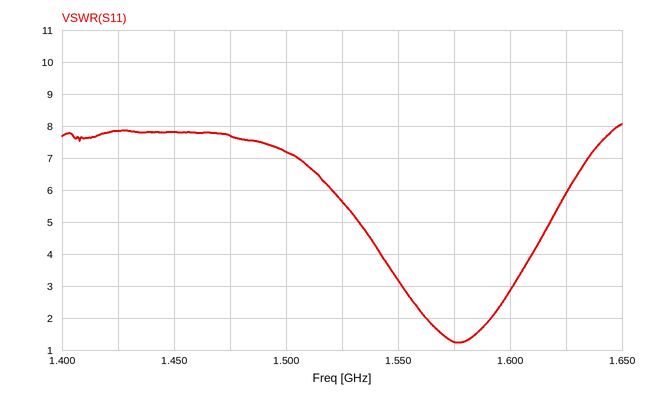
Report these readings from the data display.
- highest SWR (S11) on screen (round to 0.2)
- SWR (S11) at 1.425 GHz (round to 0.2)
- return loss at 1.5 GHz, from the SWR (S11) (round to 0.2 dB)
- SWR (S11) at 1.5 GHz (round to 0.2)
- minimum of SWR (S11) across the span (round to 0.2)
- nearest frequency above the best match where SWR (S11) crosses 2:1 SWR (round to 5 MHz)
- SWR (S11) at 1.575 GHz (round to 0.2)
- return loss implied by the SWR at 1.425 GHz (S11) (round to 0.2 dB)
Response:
8.0
7.8
2.4 dB
7.2
1.2
1.590 GHz
1.2
2.2 dB
